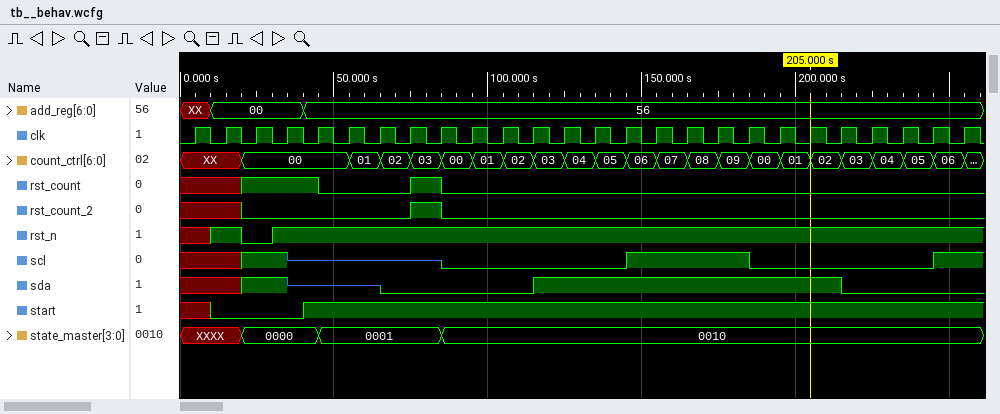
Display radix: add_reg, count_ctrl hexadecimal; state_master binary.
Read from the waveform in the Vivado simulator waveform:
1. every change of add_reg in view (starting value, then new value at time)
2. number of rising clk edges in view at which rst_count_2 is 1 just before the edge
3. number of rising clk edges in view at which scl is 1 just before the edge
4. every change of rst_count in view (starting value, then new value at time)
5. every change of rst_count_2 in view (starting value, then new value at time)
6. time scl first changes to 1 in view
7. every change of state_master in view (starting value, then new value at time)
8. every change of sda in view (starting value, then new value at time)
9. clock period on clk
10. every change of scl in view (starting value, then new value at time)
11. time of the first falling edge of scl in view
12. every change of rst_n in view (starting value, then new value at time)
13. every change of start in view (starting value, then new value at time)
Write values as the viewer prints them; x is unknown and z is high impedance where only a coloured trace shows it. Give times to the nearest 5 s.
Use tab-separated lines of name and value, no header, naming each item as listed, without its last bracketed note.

every change of add_reg in view	XX, 00 at 10 s, 56 at 40 s
number of rising clk edges in view at which rst_count_2 is 1 just before the edge	1
number of rising clk edges in view at which scl is 1 just before the edge	7
every change of rst_count in view	x, 1 at 20 s, 0 at 45 s, 1 at 75 s, 0 at 85 s
every change of rst_count_2 in view	x, 0 at 20 s, 1 at 75 s, 0 at 85 s
time scl first changes to 1 in view	20 s
every change of state_master in view	XXXX, 0000 at 20 s, 0001 at 45 s, 0010 at 85 s
every change of sda in view	x, 1 at 20 s, z at 35 s, 0 at 65 s, 1 at 115 s, 0 at 215 s
clock period on clk	10 s
every change of scl in view	x, 1 at 20 s, z at 35 s, 0 at 85 s, 1 at 145 s, 0 at 185 s, 1 at 245 s
time of the first falling edge of scl in view	185 s
every change of rst_n in view	x, 1 at 10 s, 0 at 20 s, 1 at 30 s
every change of start in view	x, 0 at 10 s, 1 at 40 s
